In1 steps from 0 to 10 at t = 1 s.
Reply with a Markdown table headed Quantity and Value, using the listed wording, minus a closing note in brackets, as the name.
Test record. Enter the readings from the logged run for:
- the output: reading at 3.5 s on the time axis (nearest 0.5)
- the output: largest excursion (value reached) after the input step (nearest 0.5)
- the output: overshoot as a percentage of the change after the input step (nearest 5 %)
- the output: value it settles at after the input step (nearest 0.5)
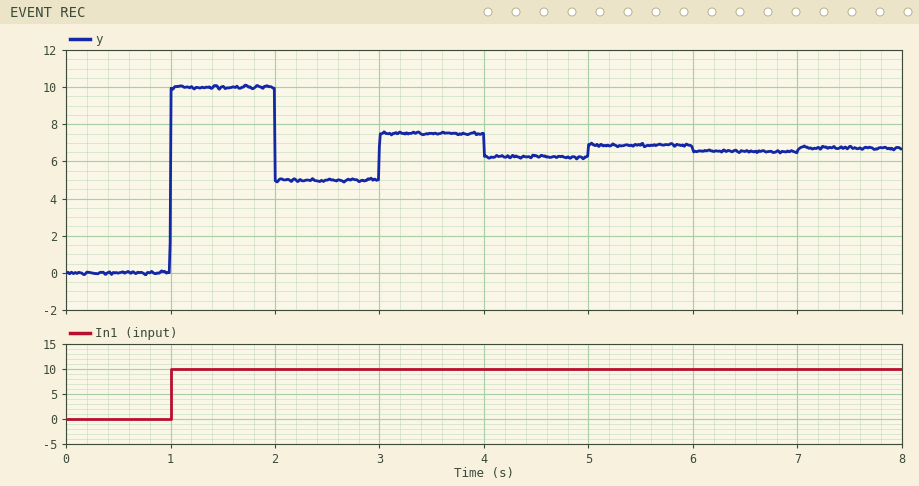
| Quantity | Value |
|---|---|
| the output: reading at 3.5 s on the time axis | 7.5 |
| the output: largest excursion (value reached) after the input step | 10.0 |
| the output: overshoot as a percentage of the change after the input step | 50 % |
| the output: value it settles at after the input step | 6.5 |
